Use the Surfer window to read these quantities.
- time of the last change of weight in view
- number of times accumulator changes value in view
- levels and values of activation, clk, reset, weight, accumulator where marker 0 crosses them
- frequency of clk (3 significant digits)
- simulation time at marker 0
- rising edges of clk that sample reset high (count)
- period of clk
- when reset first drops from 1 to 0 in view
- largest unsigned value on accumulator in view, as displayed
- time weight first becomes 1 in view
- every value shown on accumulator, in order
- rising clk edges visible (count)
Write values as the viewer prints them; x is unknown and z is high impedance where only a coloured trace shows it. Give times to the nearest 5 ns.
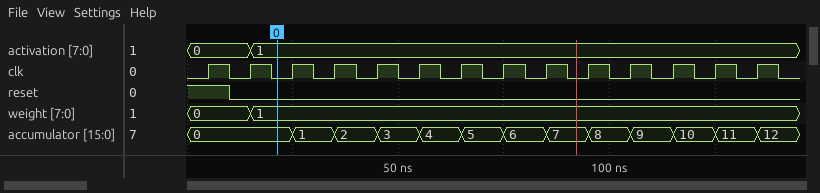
15 ns
12
activation=1, clk=0, reset=0, weight=1, accumulator=0
100 MHz
20 ns
1
10 ns
10 ns
12
15 ns
0, 1, 2, 3, 4, 5, 6, 7, 8, 9, 10, 11, 12
14
